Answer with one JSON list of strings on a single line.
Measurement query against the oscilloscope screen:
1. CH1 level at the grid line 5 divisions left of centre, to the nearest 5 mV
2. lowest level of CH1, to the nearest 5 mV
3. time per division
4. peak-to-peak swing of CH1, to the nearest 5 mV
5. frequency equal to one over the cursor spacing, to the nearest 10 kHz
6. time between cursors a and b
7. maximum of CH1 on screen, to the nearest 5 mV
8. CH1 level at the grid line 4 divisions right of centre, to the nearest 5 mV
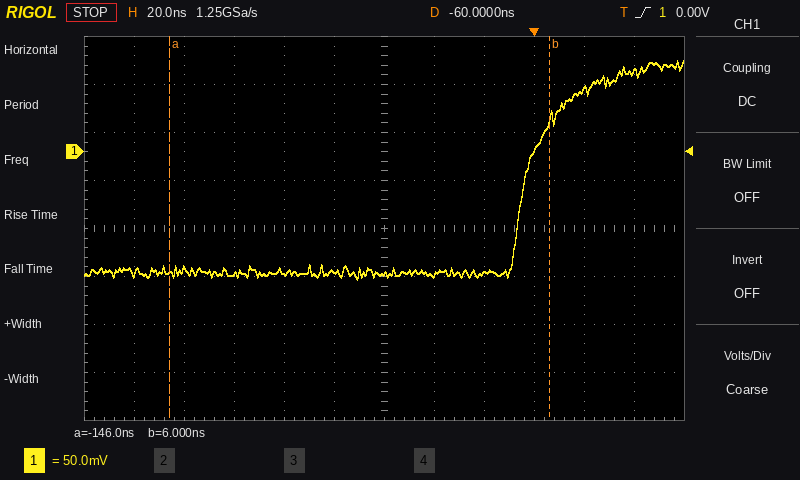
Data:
["-125 mV", "-135 mV", "20 ns", "230 mV", "6.58 MHz", "152 ns", "95 mV", "65 mV"]
